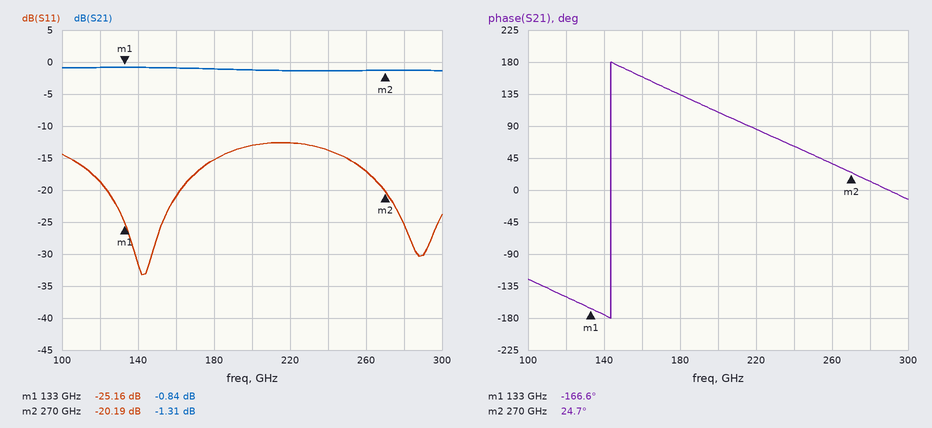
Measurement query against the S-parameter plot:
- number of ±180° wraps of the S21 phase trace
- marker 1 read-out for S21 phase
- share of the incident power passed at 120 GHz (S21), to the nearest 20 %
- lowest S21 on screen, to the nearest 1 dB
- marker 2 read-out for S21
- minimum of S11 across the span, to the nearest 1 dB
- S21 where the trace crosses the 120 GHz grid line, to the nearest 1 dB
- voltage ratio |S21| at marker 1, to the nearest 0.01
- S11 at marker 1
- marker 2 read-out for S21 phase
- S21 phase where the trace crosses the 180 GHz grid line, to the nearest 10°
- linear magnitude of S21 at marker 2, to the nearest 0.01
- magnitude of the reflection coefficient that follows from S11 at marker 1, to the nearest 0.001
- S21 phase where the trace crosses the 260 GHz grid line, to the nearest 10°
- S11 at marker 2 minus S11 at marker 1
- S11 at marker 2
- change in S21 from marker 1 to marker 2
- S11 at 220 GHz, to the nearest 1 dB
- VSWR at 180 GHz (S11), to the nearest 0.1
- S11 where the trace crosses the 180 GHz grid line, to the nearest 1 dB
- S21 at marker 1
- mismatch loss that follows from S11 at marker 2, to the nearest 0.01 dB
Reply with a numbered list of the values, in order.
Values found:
1. 1
2. -166.6°
3. 80 %
4. -1 dB
5. -1.31 dB
6. -33 dB
7. -1 dB
8. 0.91
9. -25.16 dB
10. 24.7°
11. 130°
12. 0.86
13. 0.055
14. 40°
15. 4.97 dB
16. -20.19 dB
17. -0.47 dB
18. -13 dB
19. 1.4
20. -15 dB
21. -0.84 dB
22. 0.04 dB
